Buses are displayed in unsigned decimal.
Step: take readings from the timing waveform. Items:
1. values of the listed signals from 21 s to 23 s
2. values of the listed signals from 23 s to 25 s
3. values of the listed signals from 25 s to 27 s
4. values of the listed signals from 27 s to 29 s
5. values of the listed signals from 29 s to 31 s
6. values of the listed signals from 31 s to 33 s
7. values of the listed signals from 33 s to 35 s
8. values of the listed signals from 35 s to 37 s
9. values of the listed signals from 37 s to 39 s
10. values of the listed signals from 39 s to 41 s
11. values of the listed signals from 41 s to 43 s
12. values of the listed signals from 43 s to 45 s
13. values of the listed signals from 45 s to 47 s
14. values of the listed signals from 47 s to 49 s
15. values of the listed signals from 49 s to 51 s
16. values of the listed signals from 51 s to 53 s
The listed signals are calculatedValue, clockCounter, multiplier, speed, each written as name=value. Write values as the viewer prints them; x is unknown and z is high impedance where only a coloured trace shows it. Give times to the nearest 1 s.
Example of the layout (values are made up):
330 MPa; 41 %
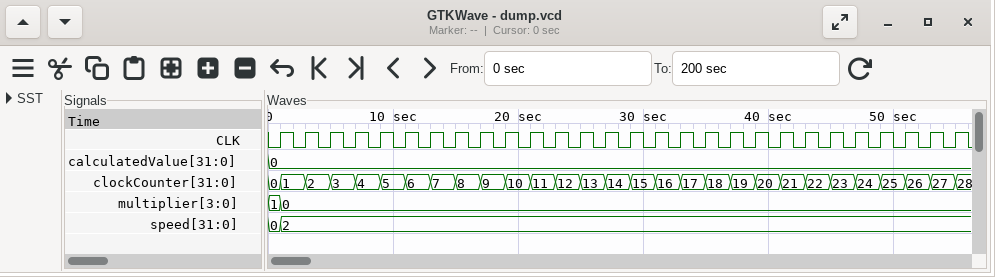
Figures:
calculatedValue=0, clockCounter=11, multiplier=0, speed=2; calculatedValue=0, clockCounter=12, multiplier=0, speed=2; calculatedValue=0, clockCounter=13, multiplier=0, speed=2; calculatedValue=0, clockCounter=14, multiplier=0, speed=2; calculatedValue=0, clockCounter=15, multiplier=0, speed=2; calculatedValue=0, clockCounter=16, multiplier=0, speed=2; calculatedValue=0, clockCounter=17, multiplier=0, speed=2; calculatedValue=0, clockCounter=18, multiplier=0, speed=2; calculatedValue=0, clockCounter=19, multiplier=0, speed=2; calculatedValue=0, clockCounter=20, multiplier=0, speed=2; calculatedValue=0, clockCounter=21, multiplier=0, speed=2; calculatedValue=0, clockCounter=22, multiplier=0, speed=2; calculatedValue=0, clockCounter=23, multiplier=0, speed=2; calculatedValue=0, clockCounter=24, multiplier=0, speed=2; calculatedValue=0, clockCounter=25, multiplier=0, speed=2; calculatedValue=0, clockCounter=26, multiplier=0, speed=2
